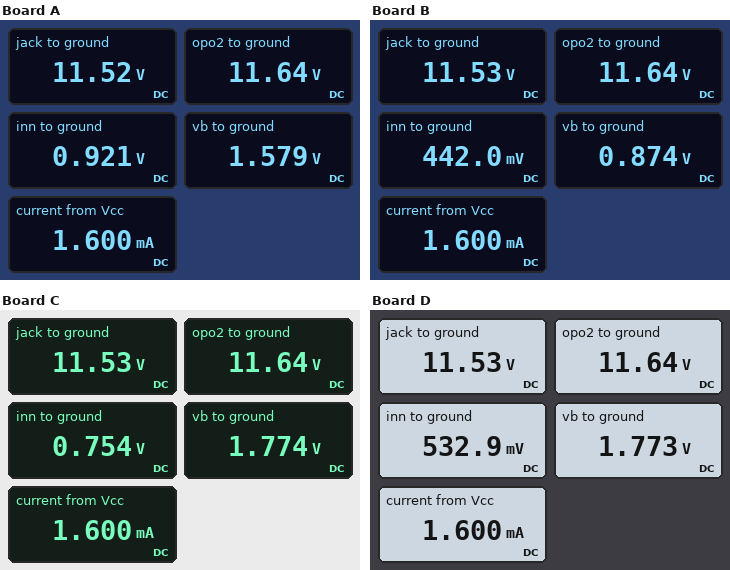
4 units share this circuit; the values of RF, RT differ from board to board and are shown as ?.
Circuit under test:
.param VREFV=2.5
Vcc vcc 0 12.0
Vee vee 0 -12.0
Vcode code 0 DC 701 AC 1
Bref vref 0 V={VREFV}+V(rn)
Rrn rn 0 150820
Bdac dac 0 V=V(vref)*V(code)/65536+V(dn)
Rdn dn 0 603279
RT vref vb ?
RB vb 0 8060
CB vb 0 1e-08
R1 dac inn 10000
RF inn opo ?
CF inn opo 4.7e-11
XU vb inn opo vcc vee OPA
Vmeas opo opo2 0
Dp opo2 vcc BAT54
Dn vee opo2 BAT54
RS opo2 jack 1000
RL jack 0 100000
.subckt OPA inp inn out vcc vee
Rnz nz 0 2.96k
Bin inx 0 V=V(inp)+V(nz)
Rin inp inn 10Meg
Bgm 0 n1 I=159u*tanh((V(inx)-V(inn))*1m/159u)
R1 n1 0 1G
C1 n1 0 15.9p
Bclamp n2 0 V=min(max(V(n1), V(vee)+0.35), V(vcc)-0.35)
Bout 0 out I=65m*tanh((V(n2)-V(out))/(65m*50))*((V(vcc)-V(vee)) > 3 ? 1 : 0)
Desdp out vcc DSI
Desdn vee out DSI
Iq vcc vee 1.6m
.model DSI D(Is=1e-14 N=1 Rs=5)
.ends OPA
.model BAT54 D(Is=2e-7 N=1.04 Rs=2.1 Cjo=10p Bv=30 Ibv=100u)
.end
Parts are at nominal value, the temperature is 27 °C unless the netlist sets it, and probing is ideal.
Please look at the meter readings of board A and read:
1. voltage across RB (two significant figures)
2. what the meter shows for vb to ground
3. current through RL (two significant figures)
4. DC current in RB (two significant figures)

1.6 V
1.579 V
120 µA
200 µA
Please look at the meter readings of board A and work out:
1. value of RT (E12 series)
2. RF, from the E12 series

4.7 kΩ
120 kΩ
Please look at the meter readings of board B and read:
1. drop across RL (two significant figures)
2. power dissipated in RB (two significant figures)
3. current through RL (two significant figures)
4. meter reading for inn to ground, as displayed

12 V
95 µW
120 µA
442.0 mV
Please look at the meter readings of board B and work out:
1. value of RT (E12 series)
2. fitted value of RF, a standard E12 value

15 kΩ
270 kΩ
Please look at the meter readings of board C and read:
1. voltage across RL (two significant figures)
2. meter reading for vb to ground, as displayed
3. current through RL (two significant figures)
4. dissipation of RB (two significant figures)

12 V
1.774 V
120 µA
390 µW
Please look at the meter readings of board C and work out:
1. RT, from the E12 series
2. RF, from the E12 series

3.3 kΩ
150 kΩ
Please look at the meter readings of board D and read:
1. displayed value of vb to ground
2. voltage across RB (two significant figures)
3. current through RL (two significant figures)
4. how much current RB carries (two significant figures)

1.773 V
1.8 V
120 µA
220 µA
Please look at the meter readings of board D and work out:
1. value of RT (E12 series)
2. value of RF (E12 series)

3.3 kΩ
220 kΩ
